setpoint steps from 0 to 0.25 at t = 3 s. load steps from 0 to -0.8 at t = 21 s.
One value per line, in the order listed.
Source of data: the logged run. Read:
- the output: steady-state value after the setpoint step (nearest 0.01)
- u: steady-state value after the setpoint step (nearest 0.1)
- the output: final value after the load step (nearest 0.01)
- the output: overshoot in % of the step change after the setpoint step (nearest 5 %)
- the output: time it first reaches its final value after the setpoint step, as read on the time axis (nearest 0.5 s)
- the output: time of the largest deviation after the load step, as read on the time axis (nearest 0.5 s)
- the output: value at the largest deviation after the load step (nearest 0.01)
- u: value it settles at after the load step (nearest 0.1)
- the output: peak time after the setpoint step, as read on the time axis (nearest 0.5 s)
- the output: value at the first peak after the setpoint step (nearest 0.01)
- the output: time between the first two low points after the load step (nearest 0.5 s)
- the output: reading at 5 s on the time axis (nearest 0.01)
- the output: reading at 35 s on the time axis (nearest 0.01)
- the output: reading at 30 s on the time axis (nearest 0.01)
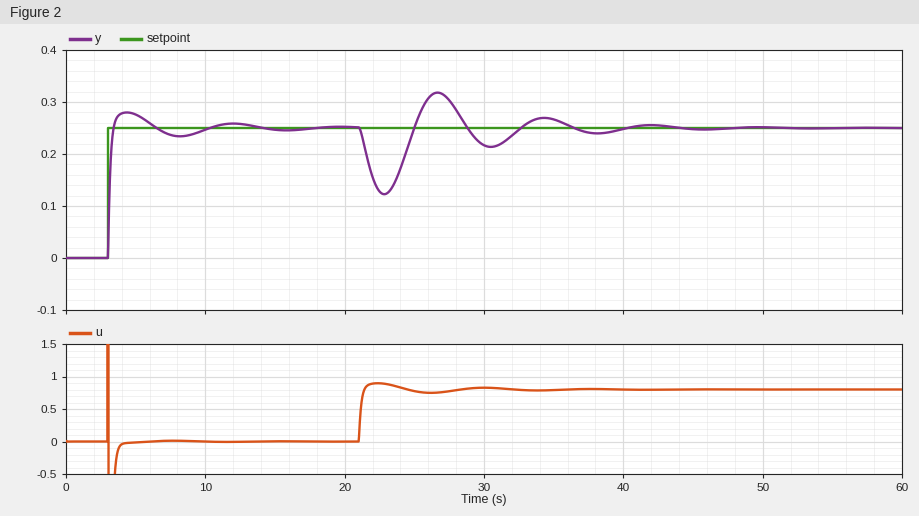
0.25
0.0
0.25
10 %
3.5 s
23.0 s
0.12
0.8
4.5 s
0.28
7.5 s
0.28
0.27
0.22
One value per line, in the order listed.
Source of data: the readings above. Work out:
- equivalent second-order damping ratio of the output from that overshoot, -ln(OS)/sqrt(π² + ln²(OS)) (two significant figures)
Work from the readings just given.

0.59
